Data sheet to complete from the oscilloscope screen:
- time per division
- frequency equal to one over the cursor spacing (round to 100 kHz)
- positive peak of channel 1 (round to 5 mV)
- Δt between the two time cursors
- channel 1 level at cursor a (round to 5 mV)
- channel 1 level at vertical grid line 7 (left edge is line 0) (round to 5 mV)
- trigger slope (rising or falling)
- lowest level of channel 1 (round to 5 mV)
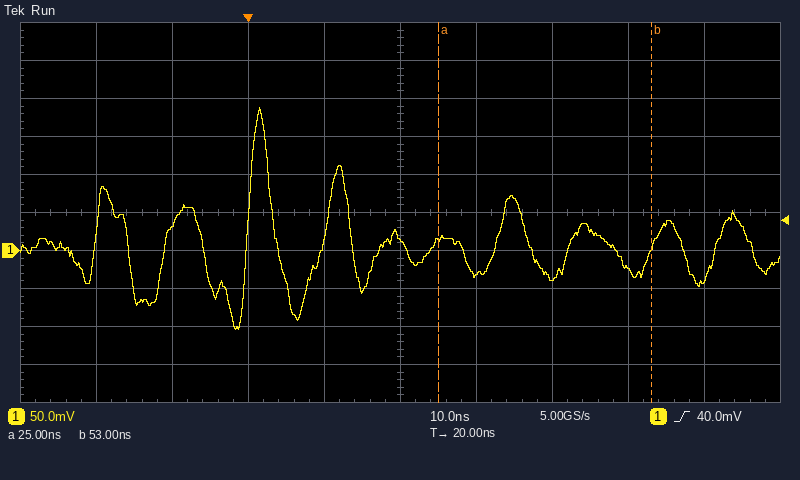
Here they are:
10 ns
35.7 MHz
190 mV
28 ns
15 mV
-35 mV
rising
-105 mV
